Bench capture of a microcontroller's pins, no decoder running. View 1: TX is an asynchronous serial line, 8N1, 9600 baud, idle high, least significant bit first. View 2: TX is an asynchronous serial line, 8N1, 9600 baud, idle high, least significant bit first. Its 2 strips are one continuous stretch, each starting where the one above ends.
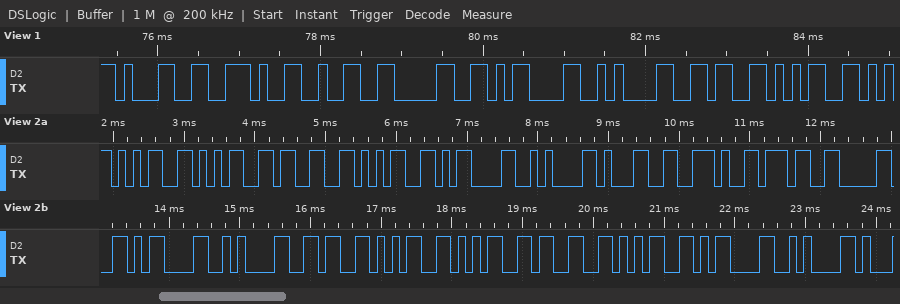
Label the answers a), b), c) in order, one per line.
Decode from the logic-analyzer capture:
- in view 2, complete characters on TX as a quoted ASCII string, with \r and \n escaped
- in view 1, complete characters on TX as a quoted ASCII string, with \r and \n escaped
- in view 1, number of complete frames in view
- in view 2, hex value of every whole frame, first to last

a) "5535\r\n1.70\r\n65535\r\n"
b) "1.20\r\n65"
c) 8
d) 35 35 33 35 0D 0A 31 2E 37 30 0D 0A 36 35 35 33 35 0D 0A
